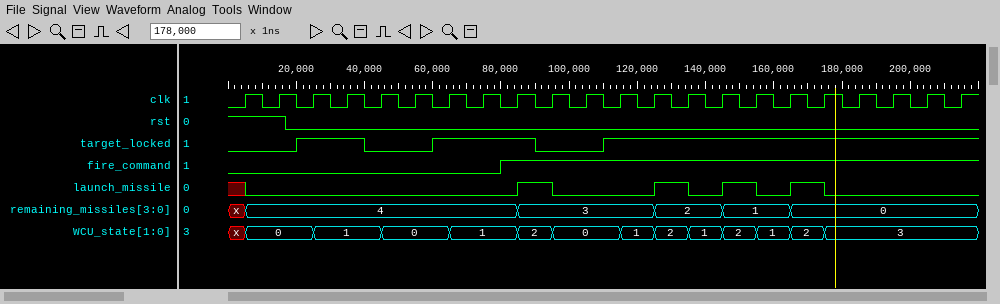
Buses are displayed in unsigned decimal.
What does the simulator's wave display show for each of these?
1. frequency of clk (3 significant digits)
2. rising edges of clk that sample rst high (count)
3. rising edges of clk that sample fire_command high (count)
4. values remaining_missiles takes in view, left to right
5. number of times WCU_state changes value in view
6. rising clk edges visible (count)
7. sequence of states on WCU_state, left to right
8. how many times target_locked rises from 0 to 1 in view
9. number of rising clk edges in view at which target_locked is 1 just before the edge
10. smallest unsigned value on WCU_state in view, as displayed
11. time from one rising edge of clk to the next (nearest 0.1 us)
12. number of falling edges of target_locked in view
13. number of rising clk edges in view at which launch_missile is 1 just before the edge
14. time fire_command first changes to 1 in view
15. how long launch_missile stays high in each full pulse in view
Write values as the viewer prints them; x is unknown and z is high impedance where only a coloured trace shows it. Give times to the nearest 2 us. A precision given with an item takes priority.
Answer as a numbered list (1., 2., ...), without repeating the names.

1. 100 kHz
2. 2
3. 14
4. x, 4, 3, 2, 1, 0
5. 13
6. 22
7. x, 0, 1, 0, 1, 2, 0, 1, 2, 1, 2, 1, 2, 3
8. 3
9. 16
10. 0
11. 10 us
12. 2
13. 4
14. 80 us
15. 10 us, 10 us, 10 us, 10 us
